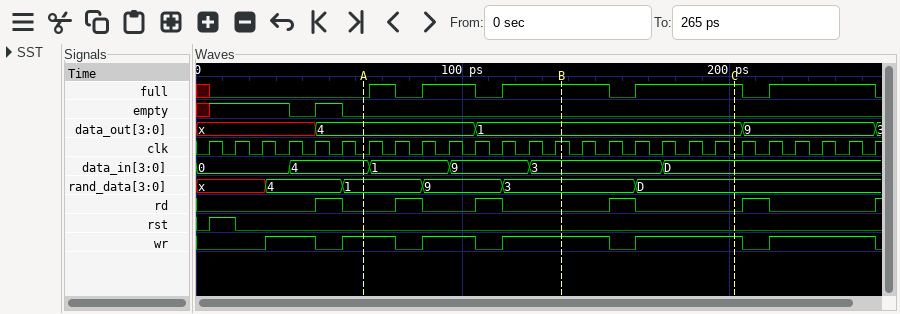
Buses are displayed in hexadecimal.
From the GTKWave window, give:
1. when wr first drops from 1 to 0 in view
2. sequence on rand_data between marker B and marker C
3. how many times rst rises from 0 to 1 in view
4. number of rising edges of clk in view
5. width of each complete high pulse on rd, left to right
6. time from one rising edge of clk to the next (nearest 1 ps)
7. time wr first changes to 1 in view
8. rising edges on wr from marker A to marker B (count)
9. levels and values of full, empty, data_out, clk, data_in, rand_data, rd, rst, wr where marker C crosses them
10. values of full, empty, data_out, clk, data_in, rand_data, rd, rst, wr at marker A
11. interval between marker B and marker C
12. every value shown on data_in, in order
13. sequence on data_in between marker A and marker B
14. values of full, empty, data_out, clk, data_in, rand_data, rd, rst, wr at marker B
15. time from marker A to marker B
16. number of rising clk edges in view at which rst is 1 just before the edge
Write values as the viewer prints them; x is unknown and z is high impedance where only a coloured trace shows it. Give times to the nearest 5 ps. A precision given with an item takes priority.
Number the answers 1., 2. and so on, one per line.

1. 45 ps
2. 3, D
3. 1
4. 26
5. 10 ps, 10 ps, 10 ps, 10 ps, 10 ps
6. 10 ps
7. 25 ps
8. 2
9. full=1, empty=0, data_out=1, clk=0, data_in=D, rand_data=D, rd=0, rst=0, wr=1
10. full=0, empty=0, data_out=4, clk=0, data_in=4, rand_data=1, rd=0, rst=0, wr=1
11. 65 ps
12. 0, 4, 1, 9, 3, D
13. 4, 1, 9, 3
14. full=1, empty=0, data_out=1, clk=1, data_in=3, rand_data=3, rd=0, rst=0, wr=1
15. 75 ps
16. 1
